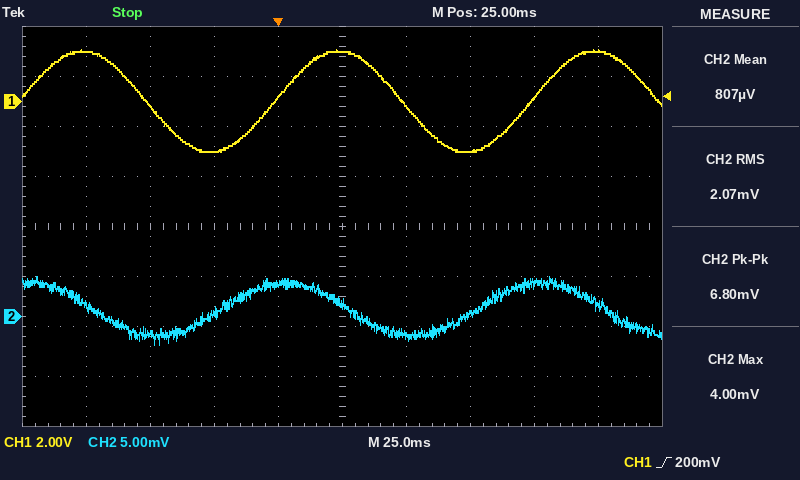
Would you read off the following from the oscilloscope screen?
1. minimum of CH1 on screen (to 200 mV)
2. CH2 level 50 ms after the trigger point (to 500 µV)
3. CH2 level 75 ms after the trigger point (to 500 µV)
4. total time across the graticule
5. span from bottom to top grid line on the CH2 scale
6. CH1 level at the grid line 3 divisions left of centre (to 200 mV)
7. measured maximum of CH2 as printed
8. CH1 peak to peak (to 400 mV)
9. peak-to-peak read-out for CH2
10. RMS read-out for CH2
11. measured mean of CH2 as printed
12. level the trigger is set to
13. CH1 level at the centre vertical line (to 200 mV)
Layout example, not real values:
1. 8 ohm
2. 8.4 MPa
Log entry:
1. -2.0 V
2. -2.0 mV
3. 0.0 mV
4. 250 ms
5. 40 mV
6. -200 mV
7. 4.00 mV
8. 4.0 V
9. 6.80 mV
10. 2.07 mV
11. 807 µV
12. 200 mV
13. 2.0 V
